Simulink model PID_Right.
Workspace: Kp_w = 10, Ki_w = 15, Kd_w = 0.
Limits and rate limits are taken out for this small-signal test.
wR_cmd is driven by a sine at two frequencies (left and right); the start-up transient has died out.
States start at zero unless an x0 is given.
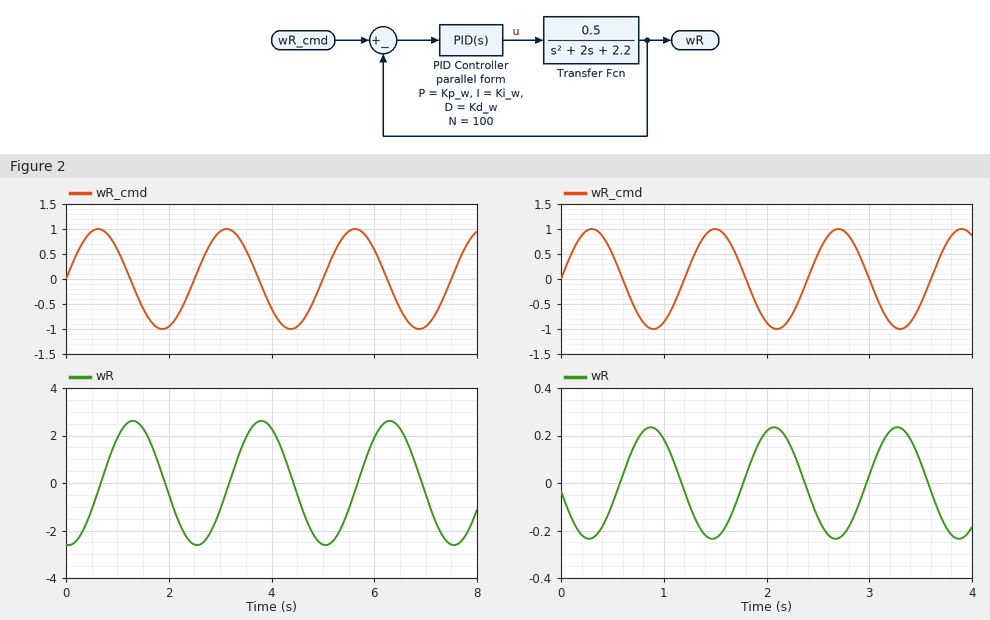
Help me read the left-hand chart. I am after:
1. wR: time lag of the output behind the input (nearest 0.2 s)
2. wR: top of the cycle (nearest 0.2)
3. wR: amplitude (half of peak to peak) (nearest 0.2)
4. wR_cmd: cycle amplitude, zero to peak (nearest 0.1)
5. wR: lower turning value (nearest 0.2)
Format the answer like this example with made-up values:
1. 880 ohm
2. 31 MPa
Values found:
1. 0.6 s
2. 2.6
3. 2.6
4. 1.0
5. -2.6
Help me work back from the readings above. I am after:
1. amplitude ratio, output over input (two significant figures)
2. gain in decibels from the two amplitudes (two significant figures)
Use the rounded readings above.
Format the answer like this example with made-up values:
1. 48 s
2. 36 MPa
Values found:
1. 2.6
2. 8.3 dB
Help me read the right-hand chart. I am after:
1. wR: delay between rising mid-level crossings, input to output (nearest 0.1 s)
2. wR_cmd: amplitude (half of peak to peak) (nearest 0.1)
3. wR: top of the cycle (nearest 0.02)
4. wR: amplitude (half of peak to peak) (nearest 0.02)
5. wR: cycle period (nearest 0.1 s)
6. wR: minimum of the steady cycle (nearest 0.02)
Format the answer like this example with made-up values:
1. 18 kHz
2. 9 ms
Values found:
1. 0.6 s
2. 1.0
3. 0.24
4. 0.24
5. 1.2 s
6. -0.24
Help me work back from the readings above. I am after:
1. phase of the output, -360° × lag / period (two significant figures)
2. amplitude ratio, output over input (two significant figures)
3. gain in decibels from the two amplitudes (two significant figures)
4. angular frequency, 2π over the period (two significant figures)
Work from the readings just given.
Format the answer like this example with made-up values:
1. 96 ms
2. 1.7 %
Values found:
1. -180°
2. 0.24
3. -12 dB
4. 5.2 rad/s
